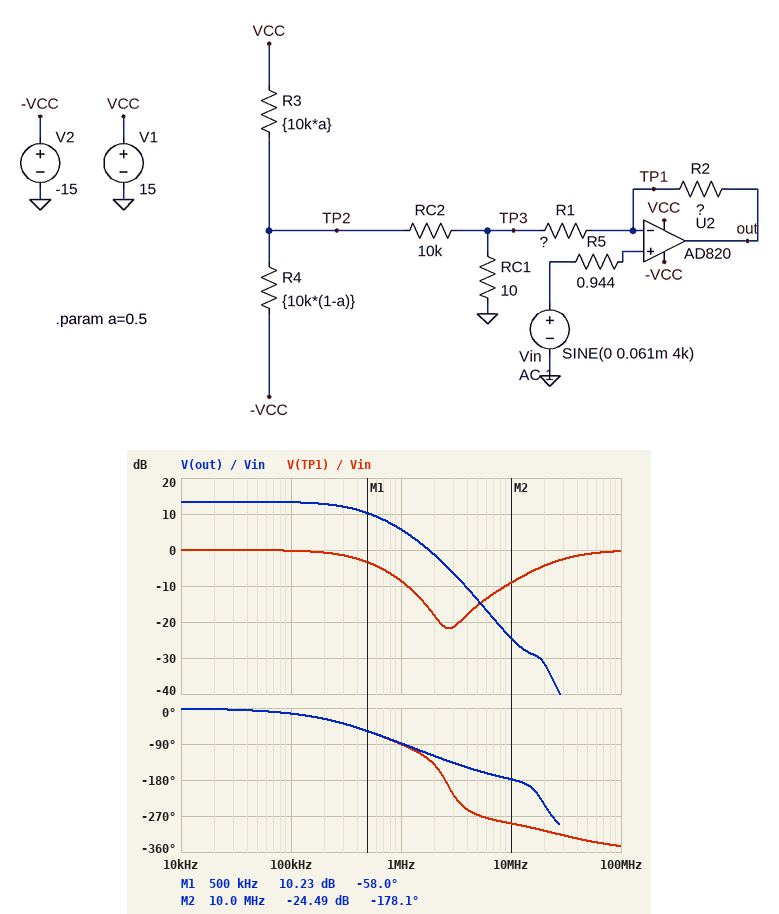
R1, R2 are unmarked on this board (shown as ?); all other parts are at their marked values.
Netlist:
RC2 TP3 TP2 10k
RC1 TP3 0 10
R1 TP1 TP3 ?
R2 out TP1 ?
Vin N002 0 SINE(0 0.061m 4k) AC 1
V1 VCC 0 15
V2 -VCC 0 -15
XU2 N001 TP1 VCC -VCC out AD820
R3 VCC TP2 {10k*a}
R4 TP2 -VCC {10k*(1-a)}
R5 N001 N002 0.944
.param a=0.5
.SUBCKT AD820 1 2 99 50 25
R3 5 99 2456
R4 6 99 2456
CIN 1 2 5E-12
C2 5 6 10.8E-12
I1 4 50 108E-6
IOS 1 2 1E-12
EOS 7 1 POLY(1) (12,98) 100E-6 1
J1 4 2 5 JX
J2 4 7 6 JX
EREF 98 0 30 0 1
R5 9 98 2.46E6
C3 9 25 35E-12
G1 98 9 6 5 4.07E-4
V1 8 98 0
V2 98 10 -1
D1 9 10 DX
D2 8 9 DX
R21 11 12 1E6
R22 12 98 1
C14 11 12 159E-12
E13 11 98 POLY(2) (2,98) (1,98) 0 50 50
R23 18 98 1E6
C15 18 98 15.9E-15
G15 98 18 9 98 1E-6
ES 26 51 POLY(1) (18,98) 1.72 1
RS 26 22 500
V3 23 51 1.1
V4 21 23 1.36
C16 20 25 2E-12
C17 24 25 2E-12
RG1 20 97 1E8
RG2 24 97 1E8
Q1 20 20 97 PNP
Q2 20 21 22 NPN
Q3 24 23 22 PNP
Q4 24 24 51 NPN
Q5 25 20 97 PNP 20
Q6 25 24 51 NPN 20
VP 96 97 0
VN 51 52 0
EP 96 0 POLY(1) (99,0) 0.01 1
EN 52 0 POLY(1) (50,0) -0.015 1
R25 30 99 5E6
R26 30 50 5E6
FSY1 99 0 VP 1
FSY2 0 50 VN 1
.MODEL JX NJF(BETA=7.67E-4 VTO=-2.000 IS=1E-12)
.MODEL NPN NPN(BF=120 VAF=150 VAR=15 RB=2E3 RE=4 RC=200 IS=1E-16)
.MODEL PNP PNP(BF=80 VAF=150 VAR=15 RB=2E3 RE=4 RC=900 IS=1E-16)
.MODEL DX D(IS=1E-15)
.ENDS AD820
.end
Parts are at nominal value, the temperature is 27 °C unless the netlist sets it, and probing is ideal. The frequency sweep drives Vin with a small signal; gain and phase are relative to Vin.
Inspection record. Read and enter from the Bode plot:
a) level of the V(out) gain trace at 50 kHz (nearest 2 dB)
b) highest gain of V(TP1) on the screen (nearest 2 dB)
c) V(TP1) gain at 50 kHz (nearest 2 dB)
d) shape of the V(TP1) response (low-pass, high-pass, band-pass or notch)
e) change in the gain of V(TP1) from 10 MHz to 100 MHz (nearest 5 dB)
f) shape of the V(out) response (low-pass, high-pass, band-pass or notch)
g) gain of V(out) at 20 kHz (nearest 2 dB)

14 dB
0 dB
0 dB
notch
10 dB
low-pass
14 dB
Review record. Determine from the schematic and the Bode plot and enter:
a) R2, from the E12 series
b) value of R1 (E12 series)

5.6 kΩ
1.5 kΩ
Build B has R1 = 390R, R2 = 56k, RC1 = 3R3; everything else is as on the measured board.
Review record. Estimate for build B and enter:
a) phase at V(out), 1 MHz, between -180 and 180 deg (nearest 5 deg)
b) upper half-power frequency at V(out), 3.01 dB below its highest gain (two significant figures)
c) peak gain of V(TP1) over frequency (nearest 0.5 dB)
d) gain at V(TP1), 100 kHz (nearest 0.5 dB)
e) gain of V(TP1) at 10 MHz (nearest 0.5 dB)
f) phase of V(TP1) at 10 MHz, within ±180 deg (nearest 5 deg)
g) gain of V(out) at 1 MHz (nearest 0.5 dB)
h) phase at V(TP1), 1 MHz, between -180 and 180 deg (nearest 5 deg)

-110 deg
13 kHz
0 dB
-18.0 dB
-18.5 dB
85 deg
5.0 dB
170 deg
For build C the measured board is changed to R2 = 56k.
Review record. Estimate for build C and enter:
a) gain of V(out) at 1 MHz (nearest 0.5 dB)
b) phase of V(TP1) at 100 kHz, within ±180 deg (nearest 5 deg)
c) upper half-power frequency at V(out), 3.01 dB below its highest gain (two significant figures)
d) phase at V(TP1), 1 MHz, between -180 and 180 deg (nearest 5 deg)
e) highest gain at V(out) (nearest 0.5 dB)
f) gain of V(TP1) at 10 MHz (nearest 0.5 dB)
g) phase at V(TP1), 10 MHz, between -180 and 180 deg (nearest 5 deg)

5.0 dB
-65 deg
50 kHz
170 deg
31.5 dB
-7.5 dB
65 deg
